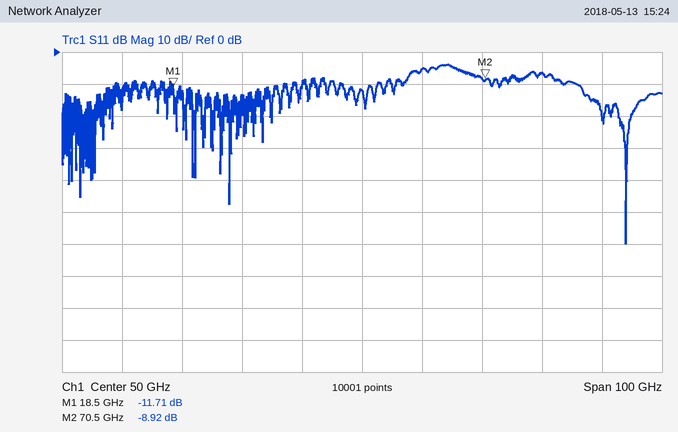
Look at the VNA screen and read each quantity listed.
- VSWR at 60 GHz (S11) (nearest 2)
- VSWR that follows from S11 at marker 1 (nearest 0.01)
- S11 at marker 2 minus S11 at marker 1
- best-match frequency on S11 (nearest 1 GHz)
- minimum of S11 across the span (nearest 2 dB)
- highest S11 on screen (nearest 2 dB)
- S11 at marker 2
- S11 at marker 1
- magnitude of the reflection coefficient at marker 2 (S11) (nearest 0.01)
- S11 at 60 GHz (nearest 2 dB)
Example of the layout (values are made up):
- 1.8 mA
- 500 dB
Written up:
- 4
- 1.70
- 2.79 dB
- 94 GHz
- -60 dB
- -4 dB
- -8.92 dB
- -11.71 dB
- 0.36
- -6 dB
